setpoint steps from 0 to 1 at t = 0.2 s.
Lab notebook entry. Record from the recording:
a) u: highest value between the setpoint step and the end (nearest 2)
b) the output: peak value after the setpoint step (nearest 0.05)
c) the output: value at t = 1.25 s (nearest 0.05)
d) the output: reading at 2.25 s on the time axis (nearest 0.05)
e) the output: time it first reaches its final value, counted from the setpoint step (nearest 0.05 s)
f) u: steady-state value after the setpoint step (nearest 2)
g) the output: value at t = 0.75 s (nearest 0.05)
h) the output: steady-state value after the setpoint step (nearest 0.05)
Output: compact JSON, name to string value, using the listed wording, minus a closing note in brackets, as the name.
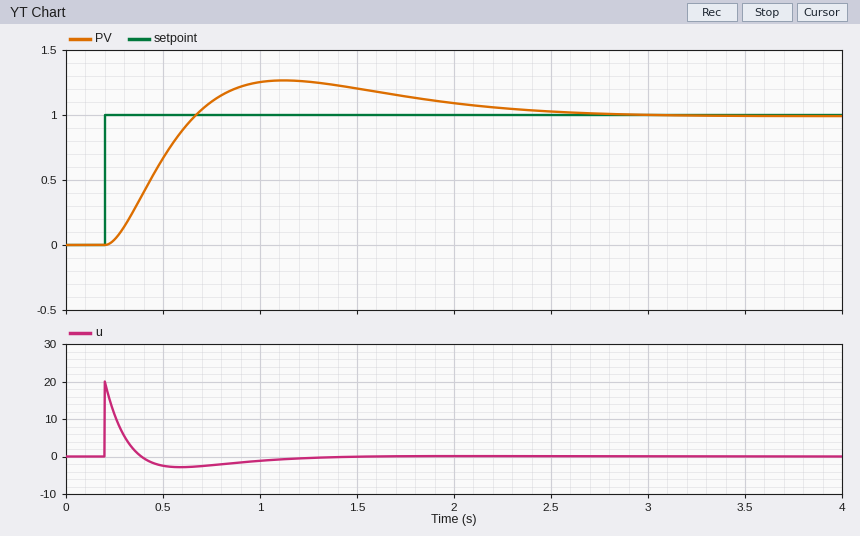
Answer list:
{"u: highest value between the setpoint step and the end": "20", "the output: peak value after the setpoint step": "1.25", "the output: value at t = 1.25 s": "1.25", "the output: reading at 2.25 s on the time axis": "1.05", "the output: time it first reaches its final value, counted from the setpoint step": "0.45 s", "u: steady-state value after the setpoint step": "0", "the output: value at t = 0.75 s": "1.10", "the output: steady-state value after the setpoint step": "1.00"}
